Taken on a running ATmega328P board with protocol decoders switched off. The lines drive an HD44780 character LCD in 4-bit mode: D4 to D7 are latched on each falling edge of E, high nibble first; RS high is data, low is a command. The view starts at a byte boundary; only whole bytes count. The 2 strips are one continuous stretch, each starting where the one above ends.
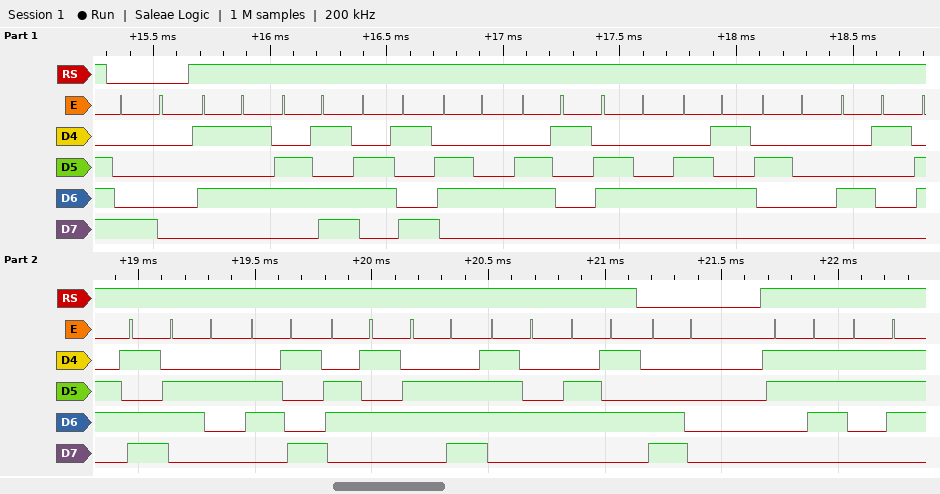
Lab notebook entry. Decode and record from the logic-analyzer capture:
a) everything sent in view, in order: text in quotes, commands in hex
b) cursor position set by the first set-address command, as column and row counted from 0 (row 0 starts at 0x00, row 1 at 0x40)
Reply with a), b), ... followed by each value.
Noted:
a) 0x80 "Umidade Ambiente" 0xC0 "77"
b) column 0, row 0
